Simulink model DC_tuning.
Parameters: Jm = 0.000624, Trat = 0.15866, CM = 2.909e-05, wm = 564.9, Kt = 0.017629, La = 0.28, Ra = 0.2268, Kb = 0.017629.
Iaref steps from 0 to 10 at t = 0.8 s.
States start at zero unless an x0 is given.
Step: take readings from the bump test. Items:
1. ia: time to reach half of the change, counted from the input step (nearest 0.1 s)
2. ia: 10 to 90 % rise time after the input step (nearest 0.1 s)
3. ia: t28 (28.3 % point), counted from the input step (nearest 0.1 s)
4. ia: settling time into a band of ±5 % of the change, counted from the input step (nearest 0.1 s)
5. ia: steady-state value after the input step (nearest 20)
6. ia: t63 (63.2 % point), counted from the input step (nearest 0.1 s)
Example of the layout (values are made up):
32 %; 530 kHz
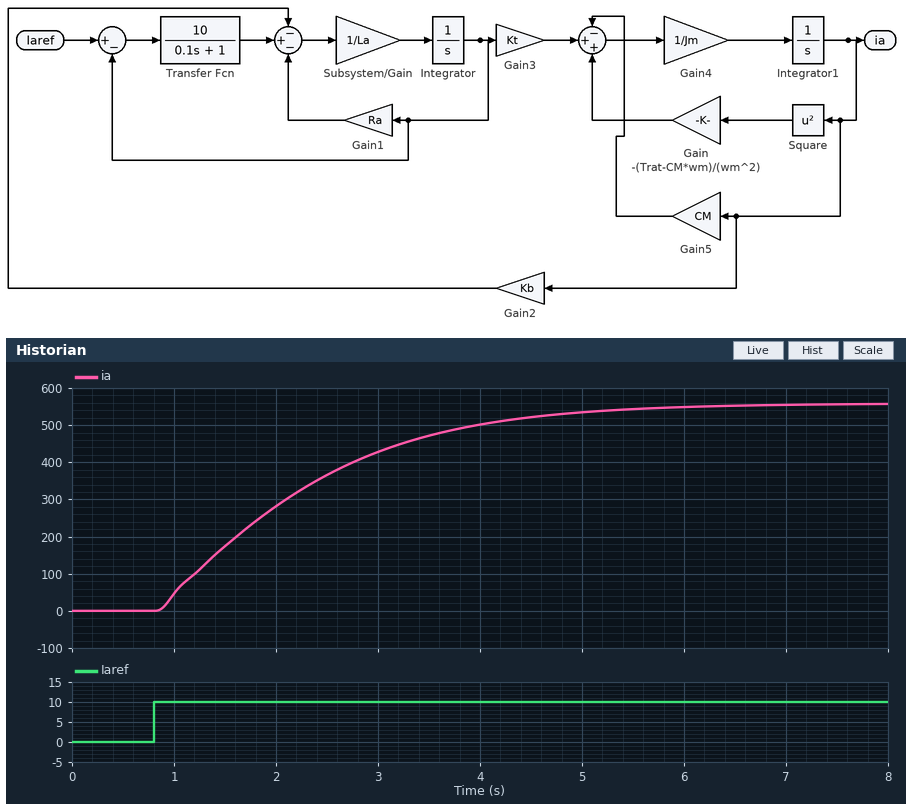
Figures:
1.2 s; 3.0 s; 0.6 s; 4.0 s; 560; 1.6 s
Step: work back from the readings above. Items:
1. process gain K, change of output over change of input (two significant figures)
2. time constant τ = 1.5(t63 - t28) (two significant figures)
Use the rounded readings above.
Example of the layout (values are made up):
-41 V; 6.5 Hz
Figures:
56; 1.5 s
